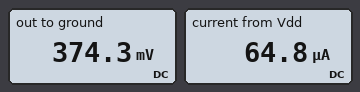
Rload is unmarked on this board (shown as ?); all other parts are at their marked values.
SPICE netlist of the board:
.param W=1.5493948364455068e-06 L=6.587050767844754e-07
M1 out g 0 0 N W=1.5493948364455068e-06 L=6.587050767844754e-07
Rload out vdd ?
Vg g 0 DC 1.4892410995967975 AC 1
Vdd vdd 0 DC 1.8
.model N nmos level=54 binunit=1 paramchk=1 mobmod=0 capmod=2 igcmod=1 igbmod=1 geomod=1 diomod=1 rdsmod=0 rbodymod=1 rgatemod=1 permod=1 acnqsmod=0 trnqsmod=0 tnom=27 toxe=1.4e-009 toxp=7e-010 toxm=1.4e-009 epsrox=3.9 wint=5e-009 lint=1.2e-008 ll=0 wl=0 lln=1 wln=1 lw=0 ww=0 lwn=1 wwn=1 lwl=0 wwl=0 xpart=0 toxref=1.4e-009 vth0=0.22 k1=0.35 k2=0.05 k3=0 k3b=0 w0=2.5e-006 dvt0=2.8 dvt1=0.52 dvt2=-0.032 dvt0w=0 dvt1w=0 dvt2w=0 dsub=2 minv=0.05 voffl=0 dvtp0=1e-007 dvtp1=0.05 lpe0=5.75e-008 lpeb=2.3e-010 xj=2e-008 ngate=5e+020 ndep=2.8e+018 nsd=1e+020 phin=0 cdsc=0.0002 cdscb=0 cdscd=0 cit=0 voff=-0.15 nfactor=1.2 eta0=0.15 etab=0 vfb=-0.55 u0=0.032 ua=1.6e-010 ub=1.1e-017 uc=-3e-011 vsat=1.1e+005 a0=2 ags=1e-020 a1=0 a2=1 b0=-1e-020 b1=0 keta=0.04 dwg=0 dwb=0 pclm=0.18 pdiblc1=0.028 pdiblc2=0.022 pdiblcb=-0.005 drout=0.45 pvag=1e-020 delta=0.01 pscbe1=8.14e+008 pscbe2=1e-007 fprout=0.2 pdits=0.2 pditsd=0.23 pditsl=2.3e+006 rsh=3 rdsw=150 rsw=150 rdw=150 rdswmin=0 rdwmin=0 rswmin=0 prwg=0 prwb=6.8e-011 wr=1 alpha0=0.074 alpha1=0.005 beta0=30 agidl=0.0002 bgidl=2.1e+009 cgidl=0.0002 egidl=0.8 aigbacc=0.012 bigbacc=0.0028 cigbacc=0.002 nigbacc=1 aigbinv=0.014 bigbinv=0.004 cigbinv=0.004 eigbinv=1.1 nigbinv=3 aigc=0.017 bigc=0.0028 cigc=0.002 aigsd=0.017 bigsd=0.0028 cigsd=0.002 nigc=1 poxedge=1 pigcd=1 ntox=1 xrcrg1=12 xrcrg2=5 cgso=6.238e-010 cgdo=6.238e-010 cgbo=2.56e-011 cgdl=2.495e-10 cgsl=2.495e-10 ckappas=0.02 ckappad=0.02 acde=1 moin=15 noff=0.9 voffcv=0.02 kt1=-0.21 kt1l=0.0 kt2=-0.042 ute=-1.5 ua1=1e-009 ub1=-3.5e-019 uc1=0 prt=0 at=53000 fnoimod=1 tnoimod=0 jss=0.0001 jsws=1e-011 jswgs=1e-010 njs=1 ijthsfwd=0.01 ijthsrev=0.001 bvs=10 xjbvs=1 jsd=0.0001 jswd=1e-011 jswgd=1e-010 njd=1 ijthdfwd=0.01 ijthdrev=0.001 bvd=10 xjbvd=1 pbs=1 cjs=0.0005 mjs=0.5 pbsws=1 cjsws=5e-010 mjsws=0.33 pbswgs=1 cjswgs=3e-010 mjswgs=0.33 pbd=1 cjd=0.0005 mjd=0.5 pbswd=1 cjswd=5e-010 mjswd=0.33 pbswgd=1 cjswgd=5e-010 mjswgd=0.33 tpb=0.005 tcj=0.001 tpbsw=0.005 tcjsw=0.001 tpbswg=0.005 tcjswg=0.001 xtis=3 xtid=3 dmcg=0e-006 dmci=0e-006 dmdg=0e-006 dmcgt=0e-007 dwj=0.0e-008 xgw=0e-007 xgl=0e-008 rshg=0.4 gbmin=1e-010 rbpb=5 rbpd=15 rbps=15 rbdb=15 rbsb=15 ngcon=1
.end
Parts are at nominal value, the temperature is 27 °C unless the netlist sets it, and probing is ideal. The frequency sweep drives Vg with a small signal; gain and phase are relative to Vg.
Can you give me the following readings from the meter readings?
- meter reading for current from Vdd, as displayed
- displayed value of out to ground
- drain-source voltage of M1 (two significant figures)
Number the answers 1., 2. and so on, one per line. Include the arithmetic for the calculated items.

1. 64.8 µA
2. 374.3 mV
3. 374.3 mV = 370 mV
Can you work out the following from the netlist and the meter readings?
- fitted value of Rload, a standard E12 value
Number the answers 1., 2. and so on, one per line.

1. 22 kΩ
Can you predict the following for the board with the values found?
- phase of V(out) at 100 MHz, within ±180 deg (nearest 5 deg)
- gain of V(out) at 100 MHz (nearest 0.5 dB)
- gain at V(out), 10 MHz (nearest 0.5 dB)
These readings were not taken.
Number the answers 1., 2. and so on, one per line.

1. 90 deg
2. -23.5 dB
3. -43.0 dB
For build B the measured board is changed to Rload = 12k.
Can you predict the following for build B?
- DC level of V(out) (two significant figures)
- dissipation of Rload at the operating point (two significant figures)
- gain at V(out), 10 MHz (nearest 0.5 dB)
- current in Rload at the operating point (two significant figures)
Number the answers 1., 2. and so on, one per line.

1. 690 mV
2. 100 µW
3. -13.5 dB
4. 92 µA
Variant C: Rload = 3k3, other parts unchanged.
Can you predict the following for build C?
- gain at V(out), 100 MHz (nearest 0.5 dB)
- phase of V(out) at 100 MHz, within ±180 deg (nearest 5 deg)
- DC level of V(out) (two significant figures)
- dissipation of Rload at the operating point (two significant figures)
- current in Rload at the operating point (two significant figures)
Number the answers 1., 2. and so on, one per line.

1. -16.0 dB
2. 170 deg
3. 1.5 V
4. 35 µW
5. 100 µA
